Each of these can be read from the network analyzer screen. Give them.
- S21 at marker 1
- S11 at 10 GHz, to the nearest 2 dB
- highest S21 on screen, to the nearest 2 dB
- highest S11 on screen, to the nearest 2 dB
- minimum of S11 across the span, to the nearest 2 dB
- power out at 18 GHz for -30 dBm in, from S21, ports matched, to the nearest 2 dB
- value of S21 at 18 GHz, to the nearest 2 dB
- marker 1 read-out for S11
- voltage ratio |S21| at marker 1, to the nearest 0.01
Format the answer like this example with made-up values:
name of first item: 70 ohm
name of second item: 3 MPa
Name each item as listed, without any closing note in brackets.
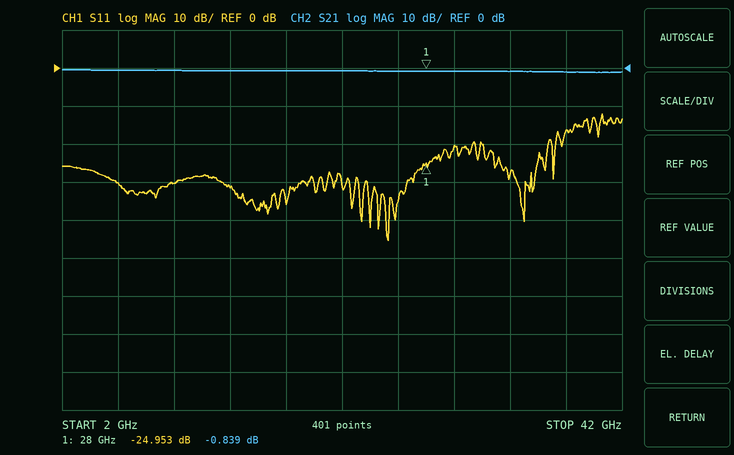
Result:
S21 at marker 1: -0.839 dB
S11 at 10 GHz, to the nearest 2 dB: -30 dB
highest S21 on screen, to the nearest 2 dB: 0 dB
highest S11 on screen, to the nearest 2 dB: -12 dB
minimum of S11 across the span, to the nearest 2 dB: -46 dB
power out at 18 GHz for -30 dBm in, from S21, ports matched, to the nearest 2 dB: -30 dBm
value of S21 at 18 GHz, to the nearest 2 dB: 0 dB
marker 1 read-out for S11: -24.953 dB
voltage ratio |S21| at marker 1, to the nearest 0.01: 0.91
